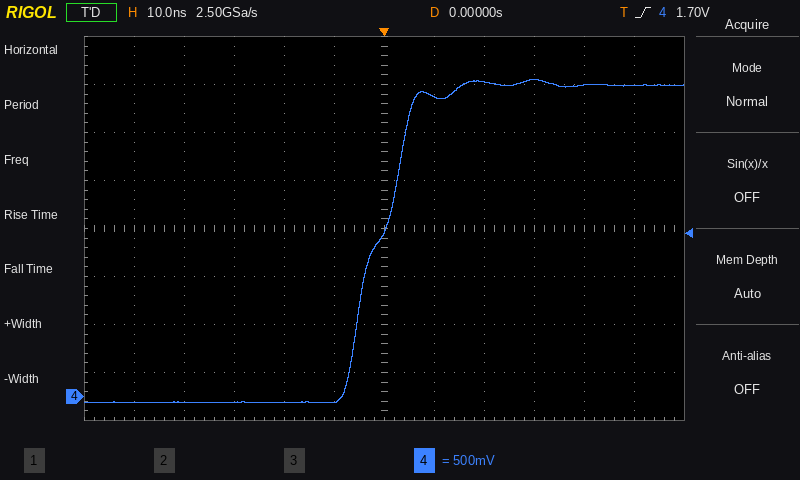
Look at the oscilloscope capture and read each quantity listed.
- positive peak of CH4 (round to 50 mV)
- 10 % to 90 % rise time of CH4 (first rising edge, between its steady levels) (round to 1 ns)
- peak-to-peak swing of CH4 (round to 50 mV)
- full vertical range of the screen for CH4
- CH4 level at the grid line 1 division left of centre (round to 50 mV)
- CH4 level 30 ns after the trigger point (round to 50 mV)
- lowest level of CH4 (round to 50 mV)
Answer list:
3.30 V
12 ns
3.35 V
4 V
-50 mV
3.30 V
-50 mV
